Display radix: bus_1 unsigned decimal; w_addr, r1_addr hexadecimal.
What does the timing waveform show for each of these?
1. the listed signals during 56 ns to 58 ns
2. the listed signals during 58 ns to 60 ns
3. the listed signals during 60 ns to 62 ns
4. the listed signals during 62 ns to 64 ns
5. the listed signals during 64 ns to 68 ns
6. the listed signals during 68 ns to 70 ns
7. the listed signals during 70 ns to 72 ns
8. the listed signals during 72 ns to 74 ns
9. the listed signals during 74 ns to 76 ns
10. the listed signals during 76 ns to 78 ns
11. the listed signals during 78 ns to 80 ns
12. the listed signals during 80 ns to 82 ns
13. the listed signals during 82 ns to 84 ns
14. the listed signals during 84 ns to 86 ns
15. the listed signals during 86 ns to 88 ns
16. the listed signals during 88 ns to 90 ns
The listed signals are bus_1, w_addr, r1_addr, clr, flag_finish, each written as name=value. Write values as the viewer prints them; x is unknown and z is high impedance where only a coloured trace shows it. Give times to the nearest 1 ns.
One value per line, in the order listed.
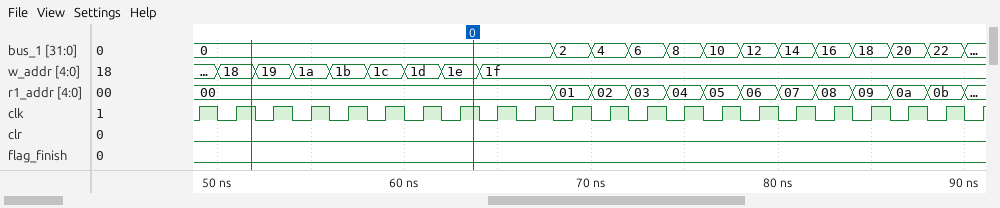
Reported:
bus_1=0, w_addr=1b, r1_addr=00, clr=0, flag_finish=0
bus_1=0, w_addr=1c, r1_addr=00, clr=0, flag_finish=0
bus_1=0, w_addr=1d, r1_addr=00, clr=0, flag_finish=0
bus_1=0, w_addr=1e, r1_addr=00, clr=0, flag_finish=0
bus_1=0, w_addr=1f, r1_addr=00, clr=0, flag_finish=0
bus_1=2, w_addr=1f, r1_addr=01, clr=0, flag_finish=0
bus_1=4, w_addr=1f, r1_addr=02, clr=0, flag_finish=0
bus_1=6, w_addr=1f, r1_addr=03, clr=0, flag_finish=0
bus_1=8, w_addr=1f, r1_addr=04, clr=0, flag_finish=0
bus_1=10, w_addr=1f, r1_addr=05, clr=0, flag_finish=0
bus_1=12, w_addr=1f, r1_addr=06, clr=0, flag_finish=0
bus_1=14, w_addr=1f, r1_addr=07, clr=0, flag_finish=0
bus_1=16, w_addr=1f, r1_addr=08, clr=0, flag_finish=0
bus_1=18, w_addr=1f, r1_addr=09, clr=0, flag_finish=0
bus_1=20, w_addr=1f, r1_addr=0a, clr=0, flag_finish=0
bus_1=22, w_addr=1f, r1_addr=0b, clr=0, flag_finish=0
